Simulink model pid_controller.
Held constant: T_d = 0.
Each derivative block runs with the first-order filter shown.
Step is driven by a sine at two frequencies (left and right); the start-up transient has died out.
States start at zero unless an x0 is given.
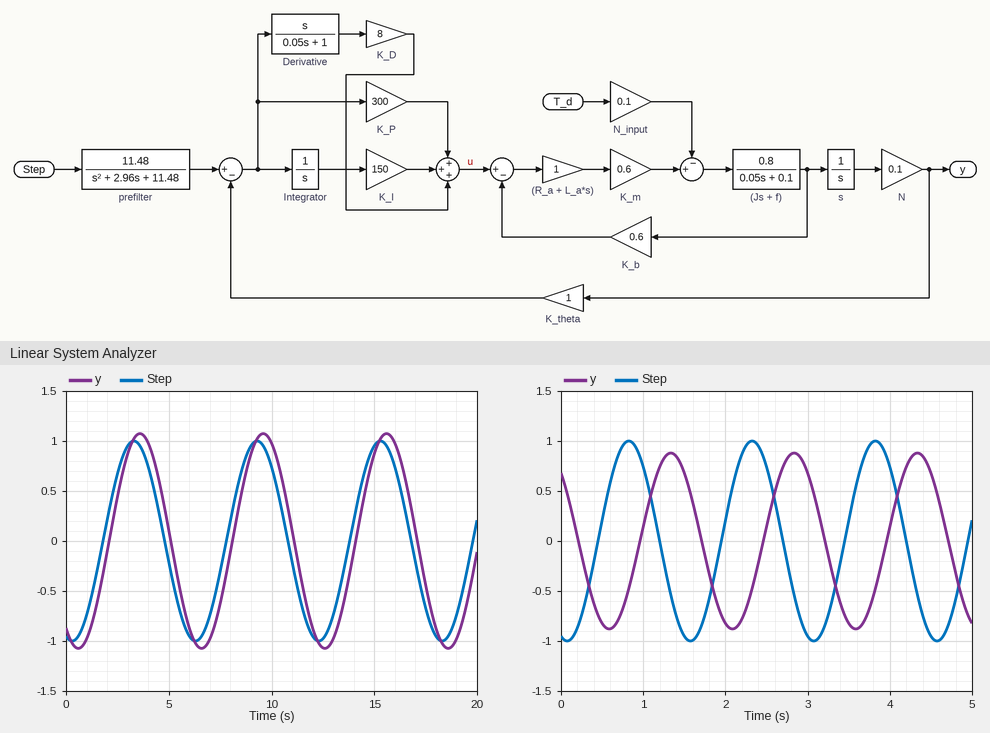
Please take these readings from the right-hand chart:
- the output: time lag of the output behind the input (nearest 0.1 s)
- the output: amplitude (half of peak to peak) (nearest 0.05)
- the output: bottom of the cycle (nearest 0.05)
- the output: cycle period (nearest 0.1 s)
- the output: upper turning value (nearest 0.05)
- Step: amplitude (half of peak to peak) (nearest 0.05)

0.5 s
0.90
-0.90
1.5 s
0.90
1.00
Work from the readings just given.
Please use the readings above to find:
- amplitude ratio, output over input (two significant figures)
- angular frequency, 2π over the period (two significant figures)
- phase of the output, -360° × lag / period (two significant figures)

0.90
4.2 rad/s
-120°
